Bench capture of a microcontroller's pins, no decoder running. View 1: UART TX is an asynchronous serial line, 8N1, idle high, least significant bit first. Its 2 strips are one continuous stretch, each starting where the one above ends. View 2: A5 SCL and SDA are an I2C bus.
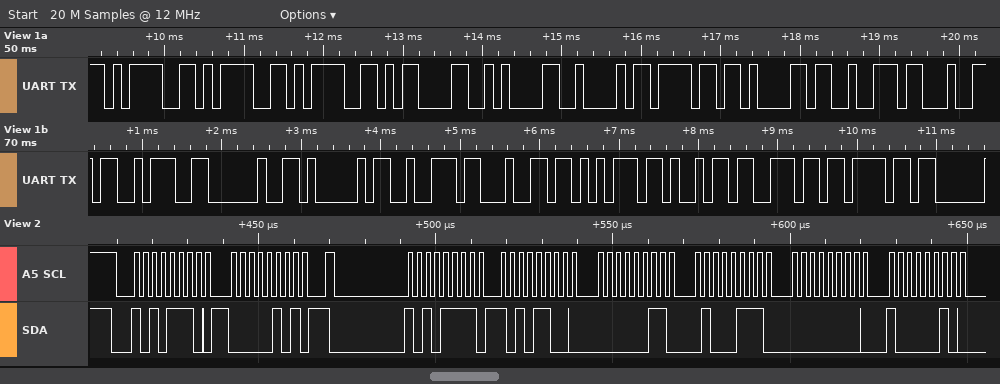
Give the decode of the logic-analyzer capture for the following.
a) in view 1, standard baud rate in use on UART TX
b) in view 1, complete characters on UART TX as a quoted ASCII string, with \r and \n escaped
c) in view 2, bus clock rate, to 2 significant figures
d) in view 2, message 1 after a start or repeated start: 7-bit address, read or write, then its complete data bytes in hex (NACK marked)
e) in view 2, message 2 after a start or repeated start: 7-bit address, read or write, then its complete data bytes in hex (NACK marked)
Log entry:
9600 baud
"===\r\nBoard: Arduino"
400 kHz
0x57 write: 05
0x57 read: AC 03 47 00 82
